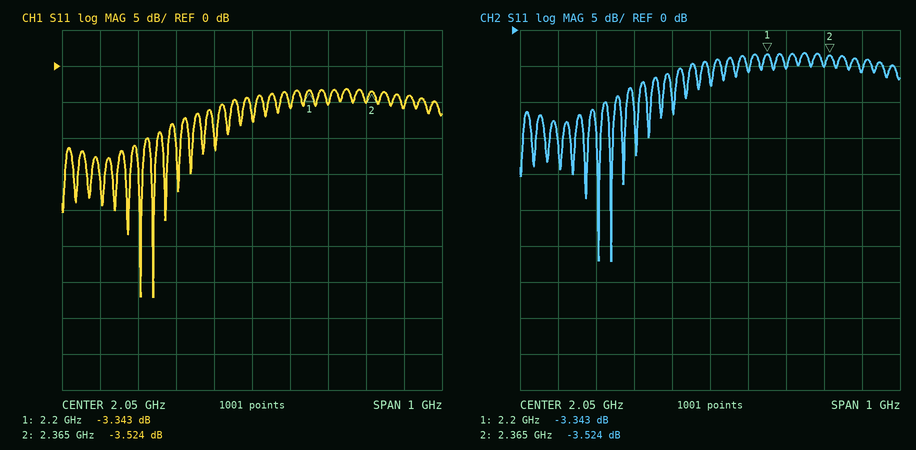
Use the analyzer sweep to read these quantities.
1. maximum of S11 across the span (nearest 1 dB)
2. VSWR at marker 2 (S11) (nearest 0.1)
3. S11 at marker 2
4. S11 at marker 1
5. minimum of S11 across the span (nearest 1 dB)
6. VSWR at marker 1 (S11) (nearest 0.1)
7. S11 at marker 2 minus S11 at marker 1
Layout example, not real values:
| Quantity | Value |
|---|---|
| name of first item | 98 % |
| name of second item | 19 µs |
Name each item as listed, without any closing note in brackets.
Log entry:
| Quantity | Value |
|---|---|
| maximum of S11 across the span | -3 dB |
| VSWR at marker 2 (S11) | 5.0 |
| S11 at marker 2 | -3.524 dB |
| S11 at marker 1 | -3.343 dB |
| minimum of S11 across the span | -32 dB |
| VSWR at marker 1 (S11) | 5.3 |
| S11 at marker 2 minus S11 at marker 1 | -0.181 dB |
